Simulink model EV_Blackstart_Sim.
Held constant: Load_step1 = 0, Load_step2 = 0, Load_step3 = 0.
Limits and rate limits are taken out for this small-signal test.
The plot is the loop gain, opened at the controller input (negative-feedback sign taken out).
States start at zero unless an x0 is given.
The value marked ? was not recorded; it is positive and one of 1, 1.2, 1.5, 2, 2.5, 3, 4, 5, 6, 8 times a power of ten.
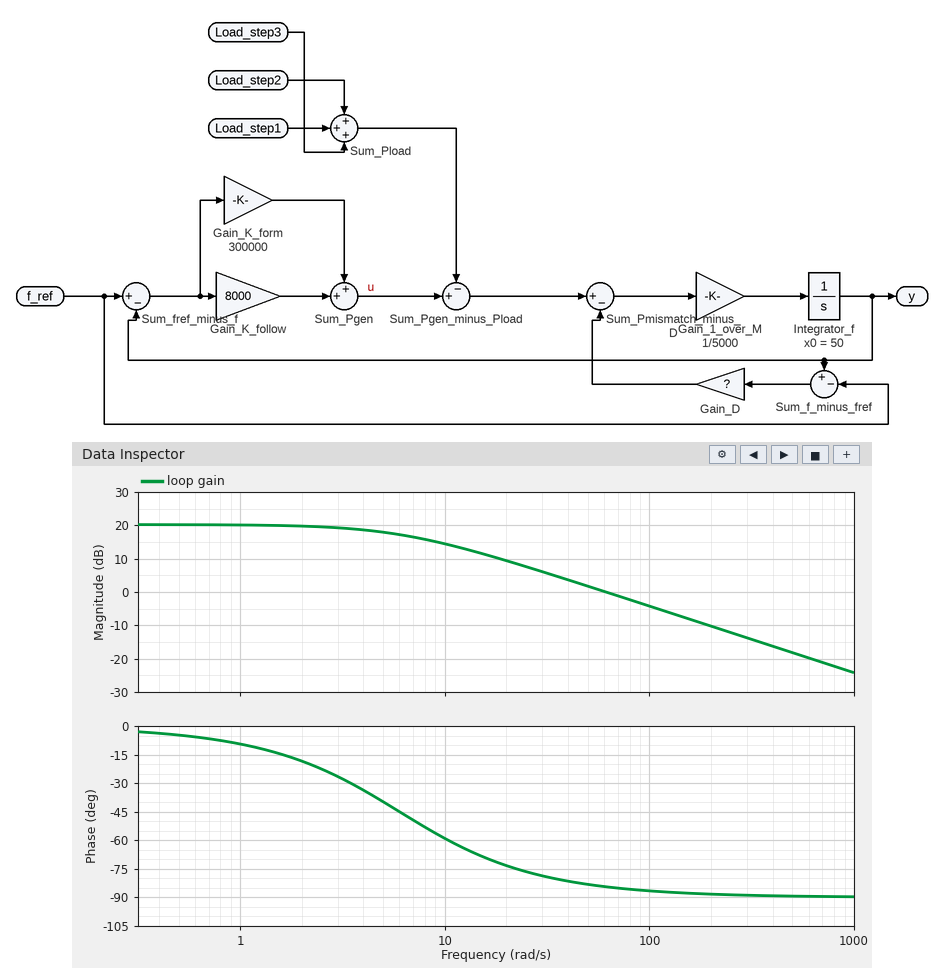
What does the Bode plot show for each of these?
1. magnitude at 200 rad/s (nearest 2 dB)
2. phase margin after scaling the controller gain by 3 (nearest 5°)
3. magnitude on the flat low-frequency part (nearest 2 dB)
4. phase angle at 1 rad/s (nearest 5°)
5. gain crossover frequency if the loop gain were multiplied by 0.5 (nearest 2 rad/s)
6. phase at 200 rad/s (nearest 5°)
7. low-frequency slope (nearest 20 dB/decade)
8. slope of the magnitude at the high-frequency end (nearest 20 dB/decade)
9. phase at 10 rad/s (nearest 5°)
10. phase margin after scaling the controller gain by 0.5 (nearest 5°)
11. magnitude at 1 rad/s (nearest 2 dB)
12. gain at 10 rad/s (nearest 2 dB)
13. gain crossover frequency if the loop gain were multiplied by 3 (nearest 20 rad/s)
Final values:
-10 dB
90°
20 dB
-10°
30 rad/s
-90°
0 dB/decade
-20 dB/decade
-60°
100°
20 dB
14 dB
180 rad/s
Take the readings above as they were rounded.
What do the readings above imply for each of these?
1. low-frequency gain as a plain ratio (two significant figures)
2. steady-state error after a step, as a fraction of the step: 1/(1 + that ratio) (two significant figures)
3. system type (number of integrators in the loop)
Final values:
10
0.091
0
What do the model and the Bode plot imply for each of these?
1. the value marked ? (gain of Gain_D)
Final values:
30000
